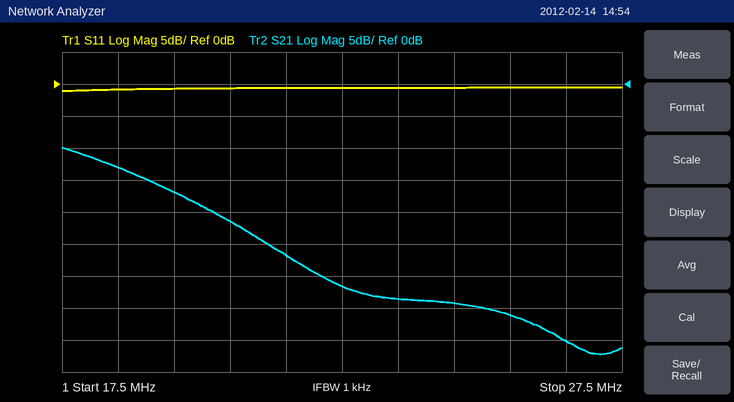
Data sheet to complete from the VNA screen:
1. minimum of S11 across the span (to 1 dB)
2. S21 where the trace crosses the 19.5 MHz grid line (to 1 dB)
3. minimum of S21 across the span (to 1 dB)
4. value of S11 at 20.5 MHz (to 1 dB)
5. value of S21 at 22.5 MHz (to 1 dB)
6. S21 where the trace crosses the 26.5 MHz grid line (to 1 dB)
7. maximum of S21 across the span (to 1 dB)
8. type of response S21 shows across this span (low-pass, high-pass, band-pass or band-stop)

-1 dB
-17 dB
-42 dB
-1 dB
-32 dB
-40 dB
-10 dB
low-pass
